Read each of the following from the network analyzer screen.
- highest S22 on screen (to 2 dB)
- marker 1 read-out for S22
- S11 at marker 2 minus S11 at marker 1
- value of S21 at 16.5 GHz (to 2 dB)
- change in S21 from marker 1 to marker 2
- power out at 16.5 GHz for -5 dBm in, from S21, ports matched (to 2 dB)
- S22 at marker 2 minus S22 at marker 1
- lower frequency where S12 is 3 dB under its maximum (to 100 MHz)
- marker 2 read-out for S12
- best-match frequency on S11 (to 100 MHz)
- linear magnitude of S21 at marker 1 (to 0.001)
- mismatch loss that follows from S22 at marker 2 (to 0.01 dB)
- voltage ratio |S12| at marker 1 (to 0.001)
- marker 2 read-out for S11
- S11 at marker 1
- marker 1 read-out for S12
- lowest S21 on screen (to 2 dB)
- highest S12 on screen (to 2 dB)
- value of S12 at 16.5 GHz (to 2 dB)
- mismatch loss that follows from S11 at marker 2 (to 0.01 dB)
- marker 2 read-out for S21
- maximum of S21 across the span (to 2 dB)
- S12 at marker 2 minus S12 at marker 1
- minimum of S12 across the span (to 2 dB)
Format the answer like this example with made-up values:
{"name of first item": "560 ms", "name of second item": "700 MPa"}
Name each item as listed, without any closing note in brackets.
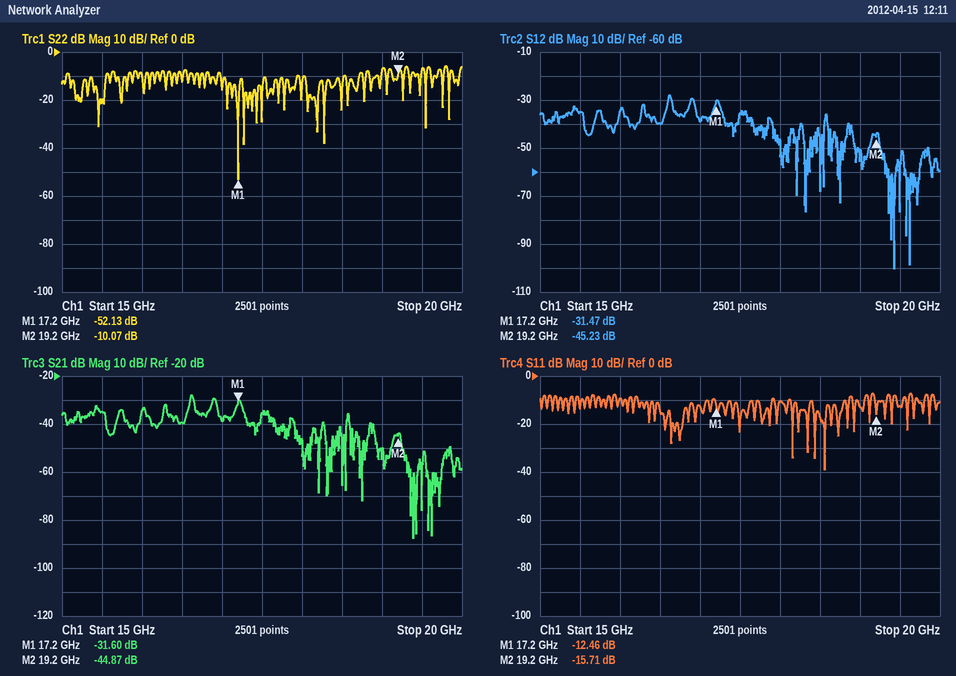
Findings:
{"highest S22 on screen": "-6 dB", "marker 1 read-out for S22": "-52.13 dB", "S11 at marker 2 minus S11 at marker 1": "-3.25 dB", "value of S21 at 16.5 GHz": "-40 dB", "change in S21 from marker 1 to marker 2": "-13.27 dB", "power out at 16.5 GHz for -5 dBm in, from S21, ports matched": "-44 dBm", "S22 at marker 2 minus S22 at marker 1": "42.06 dB", "lower frequency where S12 is 3 dB under its maximum": "16.6 GHz", "marker 2 read-out for S12": "-45.23 dB", "best-match frequency on S11": "18.6 GHz", "linear magnitude of S21 at marker 1": "0.026", "mismatch loss that follows from S22 at marker 2": "0.45 dB", "voltage ratio |S12| at marker 1": "0.027", "marker 2 read-out for S11": "-15.71 dB", "S11 at marker 1": "-12.46 dB", "marker 1 read-out for S12": "-31.47 dB", "lowest S21 on screen": "-88 dB", "highest S12 on screen": "-28 dB", "value of S12 at 16.5 GHz": "-40 dB", "mismatch loss that follows from S11 at marker 2": "0.12 dB", "marker 2 read-out for S21": "-44.87 dB", "maximum of S21 across the span": "-28 dB", "S12 at marker 2 minus S12 at marker 1": "-13.76 dB", "minimum of S12 across the span": "-100 dB"}
